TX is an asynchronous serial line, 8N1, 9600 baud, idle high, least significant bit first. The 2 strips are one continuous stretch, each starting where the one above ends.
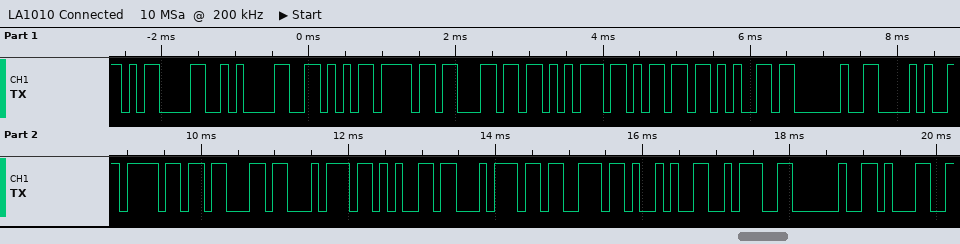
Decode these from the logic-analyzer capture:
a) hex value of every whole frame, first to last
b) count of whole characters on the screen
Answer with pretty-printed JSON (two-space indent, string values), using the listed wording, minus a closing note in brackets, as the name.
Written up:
{
  "hex value of every whole frame, first to last": "0x0D 0x0A 0x56 0x6F 0x6C 0x75 0x6D 0x65 0x20 0x28 0x6F 0x63 0x74 0x65 0x74 0x73 0x29 0x3A 0x20 0x31",
  "count of whole characters on the screen": "20"
}
